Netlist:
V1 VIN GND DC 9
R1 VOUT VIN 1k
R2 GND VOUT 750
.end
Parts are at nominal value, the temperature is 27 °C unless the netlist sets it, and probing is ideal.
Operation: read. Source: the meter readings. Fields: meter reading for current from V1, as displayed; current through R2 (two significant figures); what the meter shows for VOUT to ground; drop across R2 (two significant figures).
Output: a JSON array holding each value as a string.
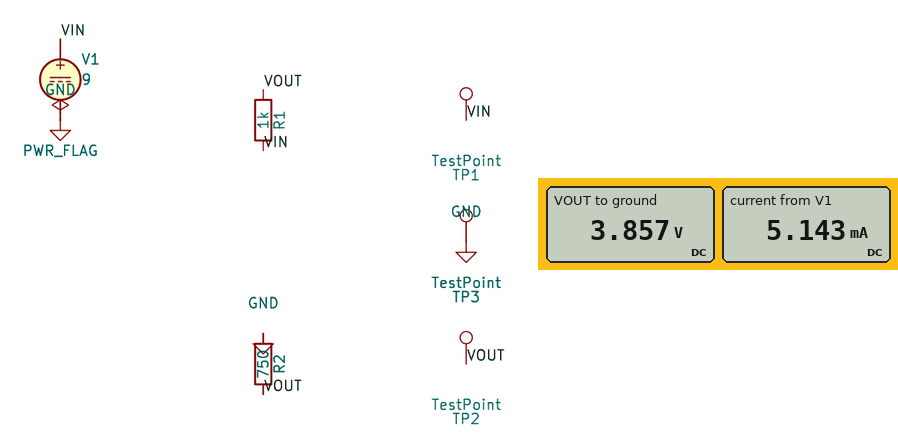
["5.143 mA", "5.1 mA", "3.857 V", "3.9 V"]
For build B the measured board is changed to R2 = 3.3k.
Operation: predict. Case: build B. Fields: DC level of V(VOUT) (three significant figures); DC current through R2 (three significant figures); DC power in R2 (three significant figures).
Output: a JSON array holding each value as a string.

["6.91 V", "2.09 mA", "14.5 mW"]
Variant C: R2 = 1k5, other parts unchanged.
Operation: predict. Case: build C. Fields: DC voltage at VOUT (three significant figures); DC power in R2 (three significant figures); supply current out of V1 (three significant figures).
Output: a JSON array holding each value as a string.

["5.40 V", "19.4 mW", "3.60 mA"]
